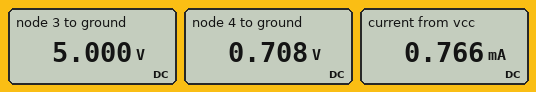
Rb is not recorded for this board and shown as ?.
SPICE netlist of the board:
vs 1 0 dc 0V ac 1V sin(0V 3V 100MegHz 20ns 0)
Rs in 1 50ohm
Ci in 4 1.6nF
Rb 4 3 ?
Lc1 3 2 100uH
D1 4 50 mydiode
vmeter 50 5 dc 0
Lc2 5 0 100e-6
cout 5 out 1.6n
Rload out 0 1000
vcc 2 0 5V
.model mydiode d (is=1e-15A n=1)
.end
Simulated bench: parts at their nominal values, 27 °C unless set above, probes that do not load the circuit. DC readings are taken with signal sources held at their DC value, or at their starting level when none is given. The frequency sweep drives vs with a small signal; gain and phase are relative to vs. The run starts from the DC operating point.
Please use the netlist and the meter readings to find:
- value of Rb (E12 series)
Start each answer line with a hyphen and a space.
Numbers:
- 5.6 kΩ
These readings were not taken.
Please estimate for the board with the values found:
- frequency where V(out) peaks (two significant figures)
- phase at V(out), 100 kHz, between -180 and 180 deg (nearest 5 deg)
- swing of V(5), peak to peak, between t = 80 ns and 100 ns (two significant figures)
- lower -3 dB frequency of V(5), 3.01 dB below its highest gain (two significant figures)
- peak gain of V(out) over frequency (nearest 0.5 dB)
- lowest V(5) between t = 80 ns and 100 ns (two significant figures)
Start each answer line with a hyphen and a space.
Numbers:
- 410 kHz
- -145 deg
- 3.9 V
- 310 kHz
- 4.0 dB
- -1.1 V
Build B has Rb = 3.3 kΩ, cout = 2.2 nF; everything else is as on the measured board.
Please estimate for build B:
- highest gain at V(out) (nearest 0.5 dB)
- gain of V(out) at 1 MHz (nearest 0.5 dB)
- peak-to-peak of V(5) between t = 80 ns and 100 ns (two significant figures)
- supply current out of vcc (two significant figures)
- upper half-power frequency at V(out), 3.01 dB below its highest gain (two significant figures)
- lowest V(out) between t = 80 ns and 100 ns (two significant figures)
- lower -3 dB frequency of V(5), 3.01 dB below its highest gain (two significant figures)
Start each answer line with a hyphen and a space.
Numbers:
- 4.5 dB
- 0.5 dB
- 4.4 V
- 1.3 mA
- 720 kHz
- -1.6 V
- 320 kHz
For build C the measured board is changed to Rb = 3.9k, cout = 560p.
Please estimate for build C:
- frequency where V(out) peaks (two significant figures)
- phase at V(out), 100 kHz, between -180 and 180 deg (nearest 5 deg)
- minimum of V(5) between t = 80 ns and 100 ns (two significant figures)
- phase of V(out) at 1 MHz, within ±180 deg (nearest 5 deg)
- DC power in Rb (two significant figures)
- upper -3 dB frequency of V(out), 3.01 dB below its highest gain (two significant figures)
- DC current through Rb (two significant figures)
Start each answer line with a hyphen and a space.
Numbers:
- 390 kHz
- -115 deg
- -1.4 V
- 30 deg
- 4.7 mW
- 670 kHz
- 1.1 mA
